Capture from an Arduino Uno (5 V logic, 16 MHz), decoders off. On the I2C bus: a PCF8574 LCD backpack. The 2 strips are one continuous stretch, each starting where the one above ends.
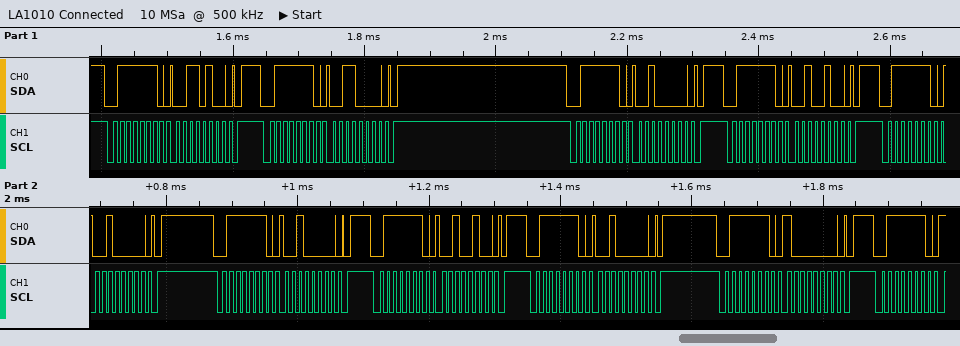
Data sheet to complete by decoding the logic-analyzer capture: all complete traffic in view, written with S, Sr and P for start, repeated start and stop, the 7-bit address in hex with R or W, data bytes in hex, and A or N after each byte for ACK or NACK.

S 3FW A 34 A P S 3FW A 30 A P S 3FW A 20 A P S 3FW A 24 A P S 3FW A 20 A P S 3FW A 20 A P S 3FW A 24 A P S 3FW A 20 A P S 3FW A 80 A P S 3FW A
